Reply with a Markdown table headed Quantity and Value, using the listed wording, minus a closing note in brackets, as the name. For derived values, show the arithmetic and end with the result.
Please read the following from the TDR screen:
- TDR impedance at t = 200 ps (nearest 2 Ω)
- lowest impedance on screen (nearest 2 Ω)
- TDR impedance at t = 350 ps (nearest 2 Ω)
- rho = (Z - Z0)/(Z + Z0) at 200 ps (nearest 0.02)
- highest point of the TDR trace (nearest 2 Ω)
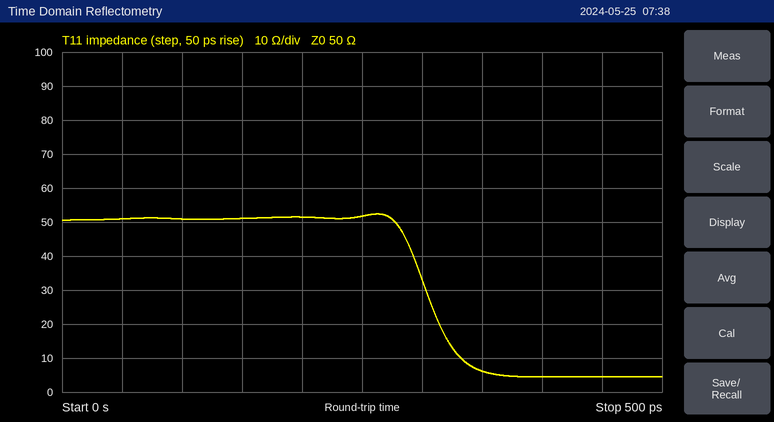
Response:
| Quantity | Value |
|---|---|
| TDR impedance at t = 200 ps | 52 Ω |
| lowest impedance on screen | 4 Ω |
| TDR impedance at t = 350 ps | 6 Ω |
| rho = (Z - Z0)/(Z + Z0) at 200 ps | (52 − 50)/(52 + 50) ≈ +0.02 |
| highest point of the TDR trace | 52 Ω |
